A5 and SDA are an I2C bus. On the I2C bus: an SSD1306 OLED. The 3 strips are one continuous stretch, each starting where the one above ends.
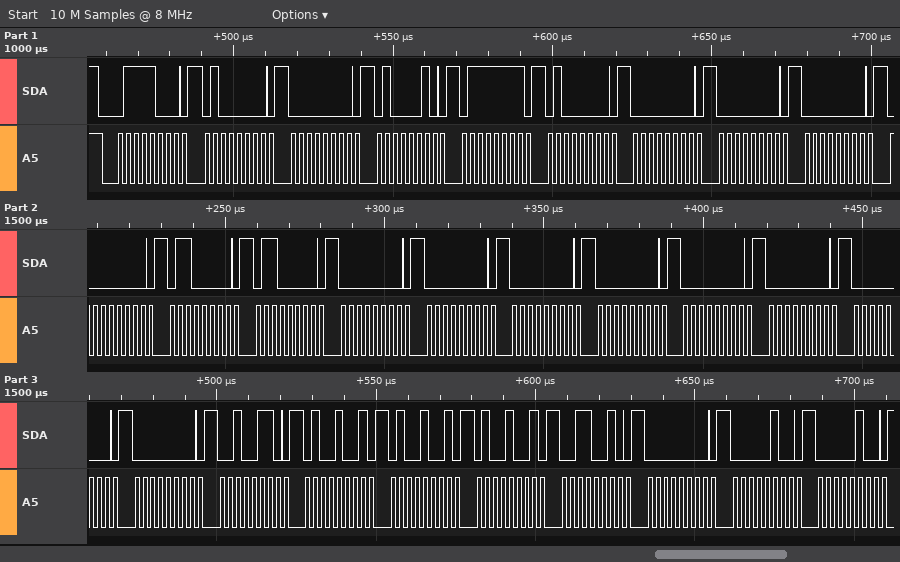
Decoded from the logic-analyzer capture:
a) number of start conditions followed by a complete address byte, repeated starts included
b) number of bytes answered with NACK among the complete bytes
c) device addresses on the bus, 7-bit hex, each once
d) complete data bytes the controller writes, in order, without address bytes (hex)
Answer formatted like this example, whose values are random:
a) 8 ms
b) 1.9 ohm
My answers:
a) 1
b) 0
c) 0x3C
d) 40 00 42 7F 40 00 00 00 00 60 60 00 00 00 00 00 00 00 00 26 49 49 49 32 00 04 04
